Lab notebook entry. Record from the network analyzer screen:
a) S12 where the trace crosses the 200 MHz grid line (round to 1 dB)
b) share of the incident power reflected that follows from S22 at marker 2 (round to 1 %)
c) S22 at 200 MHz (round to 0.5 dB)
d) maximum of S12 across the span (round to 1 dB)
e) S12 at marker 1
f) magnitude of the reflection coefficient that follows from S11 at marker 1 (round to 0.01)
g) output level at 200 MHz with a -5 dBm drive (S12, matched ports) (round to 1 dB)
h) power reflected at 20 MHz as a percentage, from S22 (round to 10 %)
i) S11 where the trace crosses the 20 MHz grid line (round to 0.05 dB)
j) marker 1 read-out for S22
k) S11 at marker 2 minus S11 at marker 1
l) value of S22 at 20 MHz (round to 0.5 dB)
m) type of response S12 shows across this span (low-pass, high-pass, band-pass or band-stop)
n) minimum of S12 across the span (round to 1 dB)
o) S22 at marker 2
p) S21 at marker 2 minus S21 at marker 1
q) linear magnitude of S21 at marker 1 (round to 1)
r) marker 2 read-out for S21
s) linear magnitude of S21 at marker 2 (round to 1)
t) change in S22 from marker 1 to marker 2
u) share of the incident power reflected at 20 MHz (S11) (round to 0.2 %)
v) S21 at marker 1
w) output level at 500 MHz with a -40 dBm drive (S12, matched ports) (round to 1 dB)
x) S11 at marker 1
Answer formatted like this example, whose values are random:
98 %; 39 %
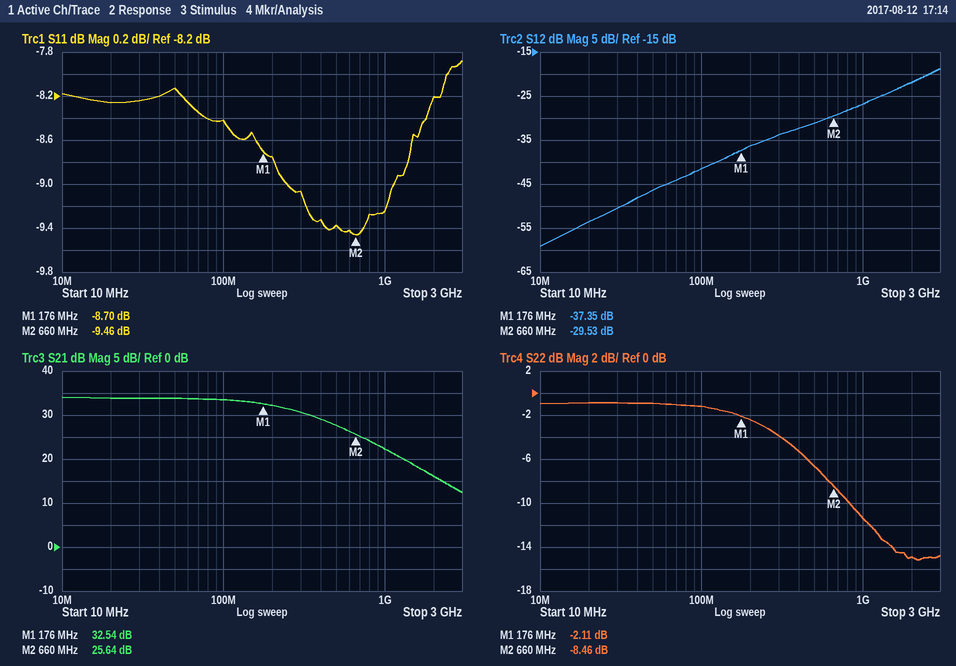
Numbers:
-36 dB; 14 %; -2.5 dB; -19 dB; -37.35 dB; 0.37; -41 dBm; 80 %; -8.25 dB; -2.11 dB; -0.76 dB; -1.0 dB; high-pass; -59 dB; -8.46 dB; -6.90 dB; 42; 25.64 dB; 19; -6.35 dB; 15.0 %; 32.54 dB; -71 dBm; -8.70 dB
